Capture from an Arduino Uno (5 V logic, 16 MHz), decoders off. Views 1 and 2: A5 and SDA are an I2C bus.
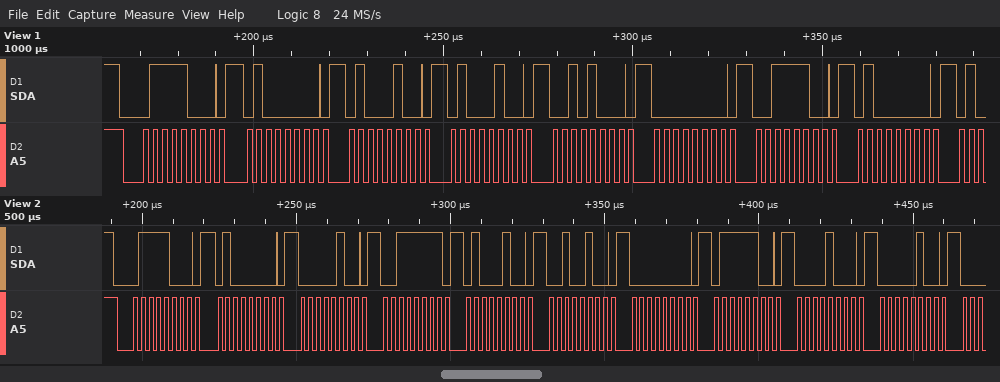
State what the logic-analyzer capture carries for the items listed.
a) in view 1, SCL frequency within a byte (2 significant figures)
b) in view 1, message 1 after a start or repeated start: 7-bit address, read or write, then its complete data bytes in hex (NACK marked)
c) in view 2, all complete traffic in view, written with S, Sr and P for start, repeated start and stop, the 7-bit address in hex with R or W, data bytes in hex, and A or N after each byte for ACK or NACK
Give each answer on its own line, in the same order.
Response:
400 kHz
0x3C write: 40 44 44 28 00 3C 40
S 3CW A 40 A 04 A 3F A 44 A 24 A 00 A 7C A 08 A 04 A
